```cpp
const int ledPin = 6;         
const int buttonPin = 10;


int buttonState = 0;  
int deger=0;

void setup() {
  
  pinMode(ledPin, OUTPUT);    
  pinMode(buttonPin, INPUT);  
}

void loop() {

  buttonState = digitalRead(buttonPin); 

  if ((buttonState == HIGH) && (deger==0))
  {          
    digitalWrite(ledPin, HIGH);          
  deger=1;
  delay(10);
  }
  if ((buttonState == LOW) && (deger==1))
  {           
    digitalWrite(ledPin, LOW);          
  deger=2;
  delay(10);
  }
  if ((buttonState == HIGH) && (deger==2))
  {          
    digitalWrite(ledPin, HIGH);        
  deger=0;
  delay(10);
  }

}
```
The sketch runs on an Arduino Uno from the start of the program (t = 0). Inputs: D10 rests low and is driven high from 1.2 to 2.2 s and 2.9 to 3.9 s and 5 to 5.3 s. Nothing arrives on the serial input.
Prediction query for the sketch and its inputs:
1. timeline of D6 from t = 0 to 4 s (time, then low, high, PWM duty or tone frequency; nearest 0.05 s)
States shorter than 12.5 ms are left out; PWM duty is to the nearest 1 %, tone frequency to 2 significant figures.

0 s low; 1.2 s high; 2.2 s low; 2.9 s high; 3.9 s low
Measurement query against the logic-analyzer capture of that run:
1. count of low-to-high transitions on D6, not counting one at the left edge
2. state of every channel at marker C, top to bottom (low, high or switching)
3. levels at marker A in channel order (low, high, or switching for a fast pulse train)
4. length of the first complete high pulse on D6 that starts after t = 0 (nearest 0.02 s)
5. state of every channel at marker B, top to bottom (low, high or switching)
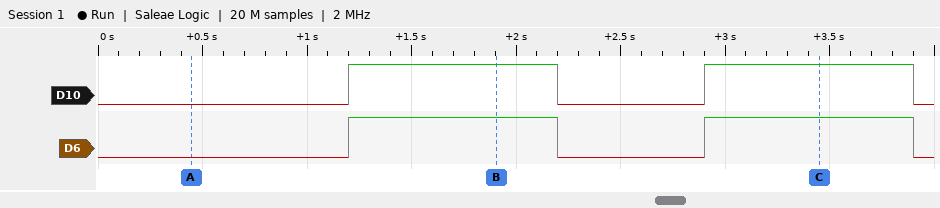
2
D10 high, D6 high
D10 low, D6 low
1.00 s
D10 high, D6 high
